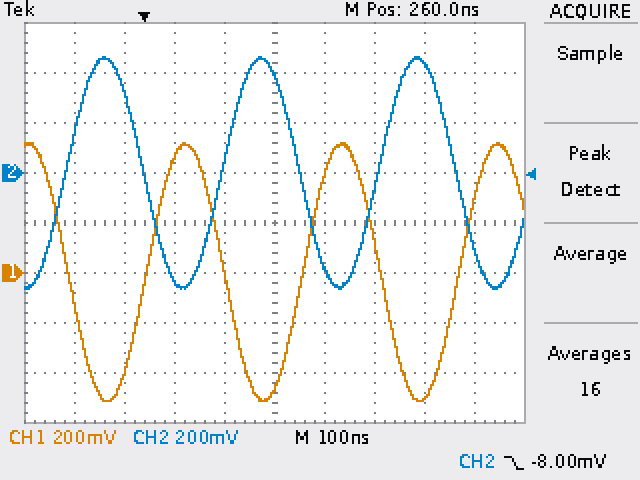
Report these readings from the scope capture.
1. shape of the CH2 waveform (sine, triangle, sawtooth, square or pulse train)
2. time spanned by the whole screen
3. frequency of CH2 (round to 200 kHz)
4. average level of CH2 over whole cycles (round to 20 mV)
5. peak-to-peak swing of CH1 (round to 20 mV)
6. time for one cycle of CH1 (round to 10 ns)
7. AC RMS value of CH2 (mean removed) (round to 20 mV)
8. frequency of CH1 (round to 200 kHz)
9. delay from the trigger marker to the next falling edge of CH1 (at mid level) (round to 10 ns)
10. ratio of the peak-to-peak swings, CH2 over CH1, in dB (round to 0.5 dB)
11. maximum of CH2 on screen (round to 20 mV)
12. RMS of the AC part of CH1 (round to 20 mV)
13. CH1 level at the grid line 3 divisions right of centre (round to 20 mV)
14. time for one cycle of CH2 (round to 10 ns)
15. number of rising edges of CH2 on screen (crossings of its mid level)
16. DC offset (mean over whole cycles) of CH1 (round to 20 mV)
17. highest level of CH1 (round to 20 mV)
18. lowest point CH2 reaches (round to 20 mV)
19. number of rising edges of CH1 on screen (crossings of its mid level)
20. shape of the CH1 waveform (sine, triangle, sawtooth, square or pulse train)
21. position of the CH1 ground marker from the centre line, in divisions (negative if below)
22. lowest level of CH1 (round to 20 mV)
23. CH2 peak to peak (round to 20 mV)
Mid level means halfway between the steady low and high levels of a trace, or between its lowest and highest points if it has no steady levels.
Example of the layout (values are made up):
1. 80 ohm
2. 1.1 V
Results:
1. sine
2. 1 µs
3. 3.2 MHz
4. 0 mV
5. 1.04 V
6. 310 ns
7. 320 mV
8. 3.2 MHz
9. 160 ns
10. -1.0 dB
11. 460 mV
12. 360 mV
13. -500 mV
14. 310 ns
15. 3
16. 0 mV
17. 520 mV
18. -460 mV
19. 3
20. sine
21. -1.0 div
22. -520 mV
23. 920 mV
